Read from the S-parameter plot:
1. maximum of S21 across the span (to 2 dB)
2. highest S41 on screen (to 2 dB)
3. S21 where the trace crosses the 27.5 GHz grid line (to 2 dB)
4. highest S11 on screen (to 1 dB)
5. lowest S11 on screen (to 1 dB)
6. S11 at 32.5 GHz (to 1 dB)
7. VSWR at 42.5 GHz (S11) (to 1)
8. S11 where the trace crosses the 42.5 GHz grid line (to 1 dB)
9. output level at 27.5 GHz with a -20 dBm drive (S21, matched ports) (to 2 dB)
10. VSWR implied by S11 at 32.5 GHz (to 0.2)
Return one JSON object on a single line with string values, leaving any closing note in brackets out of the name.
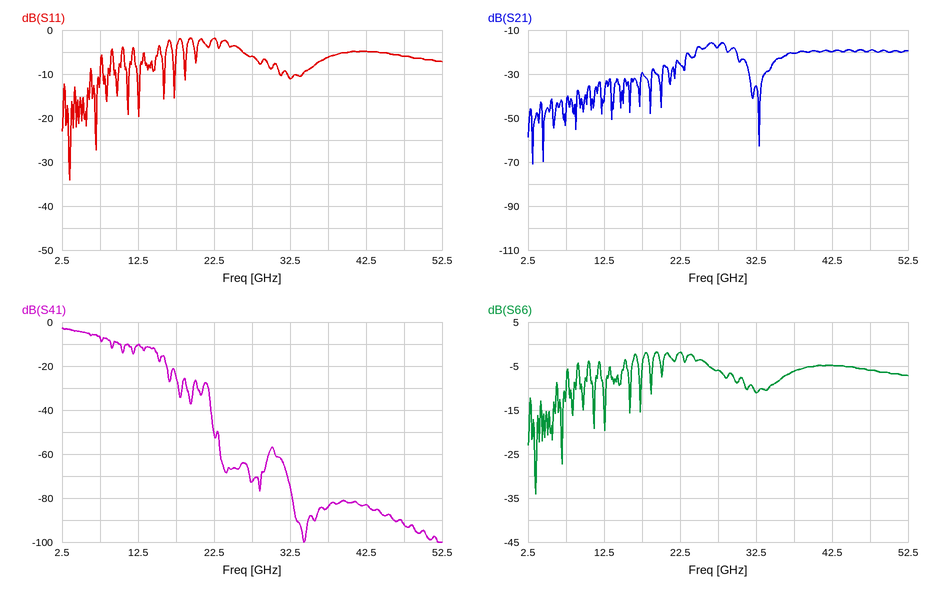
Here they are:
{"maximum of S21 across the span": "-16 dB", "highest S41 on screen": "-2 dB", "S21 where the trace crosses the 27.5 GHz grid line": "-18 dB", "highest S11 on screen": "-2 dB", "lowest S11 on screen": "-34 dB", "S11 at 32.5 GHz": "-11 dB", "VSWR at 42.5 GHz (S11)": "4", "S11 where the trace crosses the 42.5 GHz grid line": "-5 dB", "output level at 27.5 GHz with a -20 dBm drive (S21, matched ports)": "-38 dBm", "VSWR implied by S11 at 32.5 GHz": "1.8"}
